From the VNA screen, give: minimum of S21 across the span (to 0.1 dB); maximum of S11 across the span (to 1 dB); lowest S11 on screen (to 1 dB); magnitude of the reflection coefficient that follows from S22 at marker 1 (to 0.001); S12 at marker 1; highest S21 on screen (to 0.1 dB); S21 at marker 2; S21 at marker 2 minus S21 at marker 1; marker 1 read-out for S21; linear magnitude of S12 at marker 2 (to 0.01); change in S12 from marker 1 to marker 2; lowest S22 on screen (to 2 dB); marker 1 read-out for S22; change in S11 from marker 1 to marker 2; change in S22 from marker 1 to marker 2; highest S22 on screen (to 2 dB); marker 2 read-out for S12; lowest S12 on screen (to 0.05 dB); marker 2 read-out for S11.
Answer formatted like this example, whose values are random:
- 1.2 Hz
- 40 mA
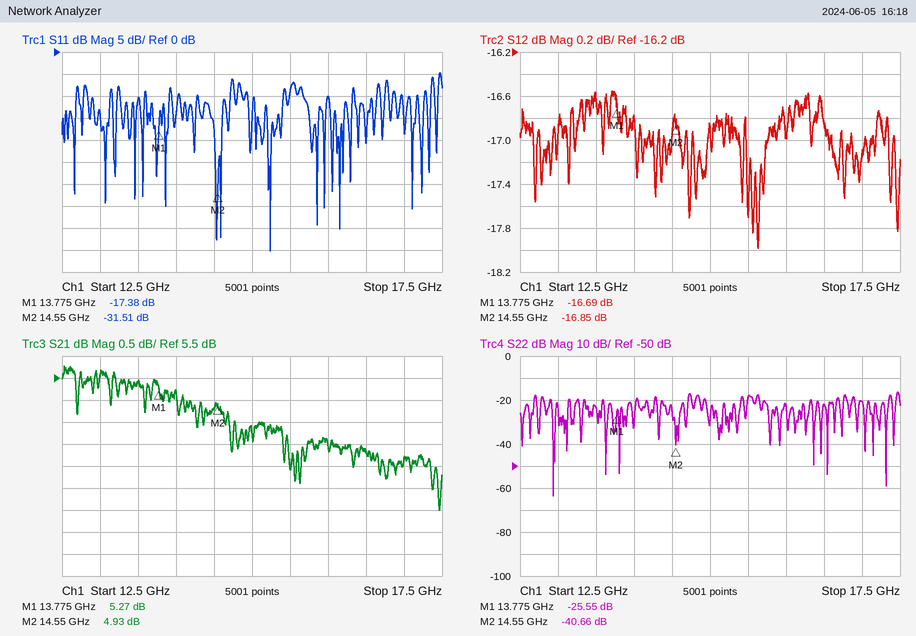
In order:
- 2.5 dB
- -5 dB
- -45 dB
- 0.053
- -16.69 dB
- 5.8 dB
- 4.93 dB
- -0.34 dB
- 5.27 dB
- 0.14
- -0.16 dB
- -64 dB
- -25.55 dB
- -14.13 dB
- -15.11 dB
- -16 dB
- -16.85 dB
- -18.00 dB
- -31.51 dB
